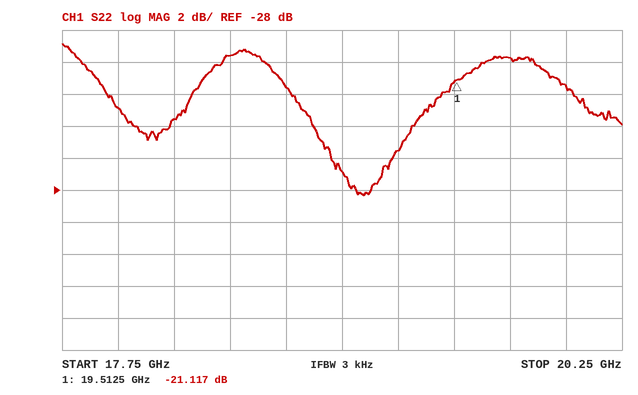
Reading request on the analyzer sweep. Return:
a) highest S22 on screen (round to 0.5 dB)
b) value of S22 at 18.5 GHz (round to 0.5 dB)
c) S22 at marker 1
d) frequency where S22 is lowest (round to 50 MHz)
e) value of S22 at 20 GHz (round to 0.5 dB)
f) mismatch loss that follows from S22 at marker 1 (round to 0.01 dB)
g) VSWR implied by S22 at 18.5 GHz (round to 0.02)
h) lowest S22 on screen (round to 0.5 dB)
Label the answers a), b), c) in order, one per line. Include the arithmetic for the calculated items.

a) -19.0 dB
b) -19.5 dB
c) -21.117 dB
d) 19.10 GHz
e) -21.5 dB
f) −10 log10(1 − 10^(-21.117/10)) ≈ 0.03 dB
g) |Γ| = 10^(-19.5/20) = 0.1059; VSWR = (1 + 0.1059)/(1 − 0.1059) ≈ 1.24
h) -28.5 dB
